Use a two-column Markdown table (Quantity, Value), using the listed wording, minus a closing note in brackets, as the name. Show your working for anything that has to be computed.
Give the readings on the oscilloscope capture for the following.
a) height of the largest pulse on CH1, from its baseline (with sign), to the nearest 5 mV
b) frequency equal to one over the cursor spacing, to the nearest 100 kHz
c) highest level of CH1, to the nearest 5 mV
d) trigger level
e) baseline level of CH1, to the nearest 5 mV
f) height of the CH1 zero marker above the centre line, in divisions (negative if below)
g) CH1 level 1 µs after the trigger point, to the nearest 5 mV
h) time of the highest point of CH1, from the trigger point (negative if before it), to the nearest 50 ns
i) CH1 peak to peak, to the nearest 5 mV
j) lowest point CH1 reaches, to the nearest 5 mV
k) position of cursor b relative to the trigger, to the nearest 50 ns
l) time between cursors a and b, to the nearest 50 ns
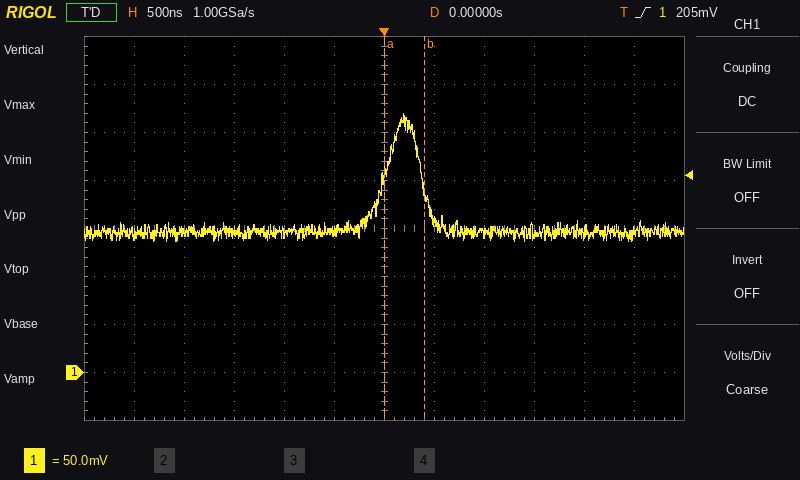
| Quantity | Value |
|---|---|
| height of the largest pulse on CH1, from its baseline (with sign), to the nearest 5 mV | 270 mV − (145 mV) = +125 mV |
| frequency equal to one over the cursor spacing, to the nearest 100 kHz | 1 / 400 ns ≈ 2.5 MHz |
| highest level of CH1, to the nearest 5 mV | 270 mV |
| trigger level | 205 mV |
| baseline level of CH1, to the nearest 5 mV | 145 mV |
| height of the CH1 zero marker above the centre line, in divisions | -3.0 div |
| CH1 level 1 µs after the trigger point, to the nearest 5 mV | 145 mV |
| time of the highest point of CH1, from the trigger point (negative if before it), to the nearest 50 ns | +200 ns |
| CH1 peak to peak, to the nearest 5 mV | 270 mV − (135 mV) = 135 mV |
| lowest point CH1 reaches, to the nearest 5 mV | 135 mV |
| position of cursor b relative to the trigger, to the nearest 50 ns | +400 ns |
| time between cursors a and b, to the nearest 50 ns | 400 ns |
